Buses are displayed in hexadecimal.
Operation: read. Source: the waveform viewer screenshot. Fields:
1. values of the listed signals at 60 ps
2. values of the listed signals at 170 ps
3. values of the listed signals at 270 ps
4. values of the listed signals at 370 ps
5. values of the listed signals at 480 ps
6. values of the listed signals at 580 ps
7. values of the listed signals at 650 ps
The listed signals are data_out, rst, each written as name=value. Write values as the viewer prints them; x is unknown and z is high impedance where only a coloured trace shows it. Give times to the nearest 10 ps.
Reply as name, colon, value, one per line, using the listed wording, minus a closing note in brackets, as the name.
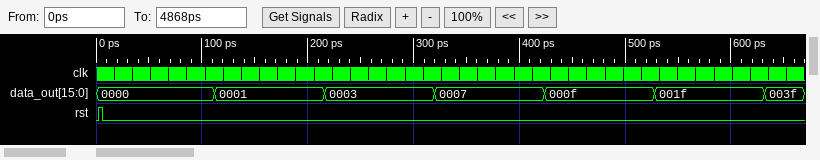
values of the listed signals at 60 ps: data_out=0000, rst=0
values of the listed signals at 170 ps: data_out=0001, rst=0
values of the listed signals at 270 ps: data_out=0003, rst=0
values of the listed signals at 370 ps: data_out=0007, rst=0
values of the listed signals at 480 ps: data_out=000f, rst=0
values of the listed signals at 580 ps: data_out=001f, rst=0
values of the listed signals at 650 ps: data_out=003f, rst=0
